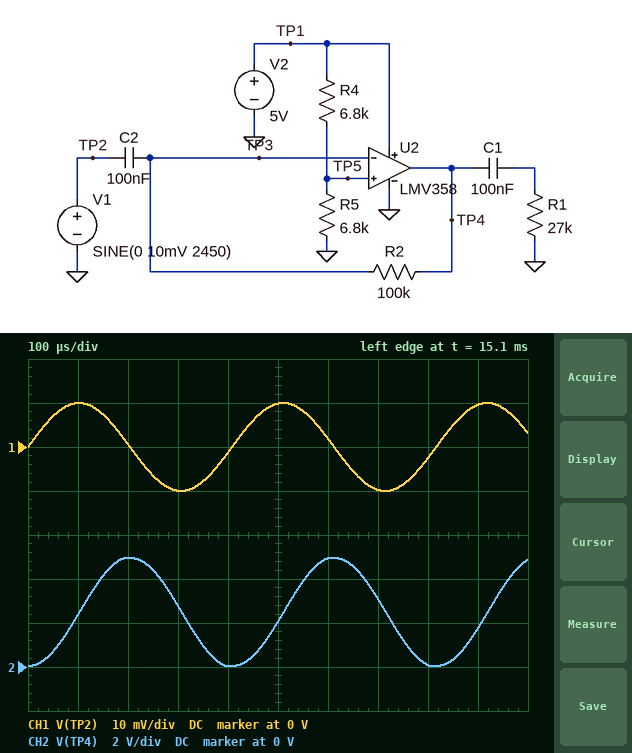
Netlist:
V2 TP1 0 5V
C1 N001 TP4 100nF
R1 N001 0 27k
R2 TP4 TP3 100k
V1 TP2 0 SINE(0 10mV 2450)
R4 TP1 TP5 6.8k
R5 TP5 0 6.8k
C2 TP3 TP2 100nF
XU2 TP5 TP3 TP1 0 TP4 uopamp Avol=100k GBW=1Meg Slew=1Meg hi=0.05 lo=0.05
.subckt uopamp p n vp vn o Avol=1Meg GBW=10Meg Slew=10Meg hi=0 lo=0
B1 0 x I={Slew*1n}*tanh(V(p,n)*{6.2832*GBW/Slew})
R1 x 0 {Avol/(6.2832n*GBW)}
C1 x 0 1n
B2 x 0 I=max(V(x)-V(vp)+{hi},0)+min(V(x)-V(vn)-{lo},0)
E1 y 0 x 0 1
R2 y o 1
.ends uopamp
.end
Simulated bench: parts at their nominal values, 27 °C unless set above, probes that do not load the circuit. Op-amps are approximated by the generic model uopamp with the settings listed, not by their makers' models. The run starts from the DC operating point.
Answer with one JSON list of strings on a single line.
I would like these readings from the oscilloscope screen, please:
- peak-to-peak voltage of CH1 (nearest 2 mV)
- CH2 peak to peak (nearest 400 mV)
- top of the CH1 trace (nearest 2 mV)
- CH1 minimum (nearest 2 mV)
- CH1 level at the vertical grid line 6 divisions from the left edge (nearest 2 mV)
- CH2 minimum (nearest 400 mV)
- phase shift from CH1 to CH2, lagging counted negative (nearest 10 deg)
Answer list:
["20 mV", "4.8 V", "10 mV", "-10 mV", "2 mV", "0 V", "-90 deg"]
